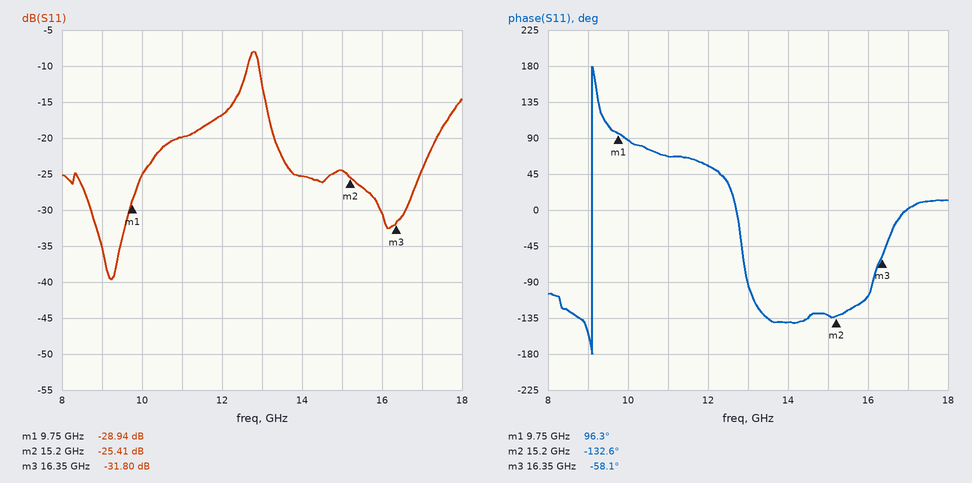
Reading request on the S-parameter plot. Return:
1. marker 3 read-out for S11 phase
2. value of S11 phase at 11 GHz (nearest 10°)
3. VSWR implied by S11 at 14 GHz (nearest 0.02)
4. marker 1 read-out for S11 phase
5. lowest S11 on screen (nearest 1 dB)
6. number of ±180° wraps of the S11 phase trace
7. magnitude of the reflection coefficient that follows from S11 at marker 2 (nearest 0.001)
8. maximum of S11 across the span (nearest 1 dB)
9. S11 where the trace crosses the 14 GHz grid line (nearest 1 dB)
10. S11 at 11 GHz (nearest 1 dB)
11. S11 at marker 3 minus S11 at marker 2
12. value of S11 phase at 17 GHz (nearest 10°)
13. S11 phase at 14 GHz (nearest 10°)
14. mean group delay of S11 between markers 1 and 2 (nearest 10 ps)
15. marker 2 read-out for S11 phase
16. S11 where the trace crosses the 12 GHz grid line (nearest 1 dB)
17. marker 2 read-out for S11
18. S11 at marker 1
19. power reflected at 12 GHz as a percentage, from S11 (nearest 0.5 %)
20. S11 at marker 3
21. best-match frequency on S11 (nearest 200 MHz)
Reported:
-58.1°
70°
1.12
96.3°
-40 dB
1
0.054
-8 dB
-25 dB
-20 dB
-6.39 dB
0°
-140°
120 ps
-132.6°
-17 dB
-25.41 dB
-28.94 dB
2.0 %
-31.80 dB
9.2 GHz
